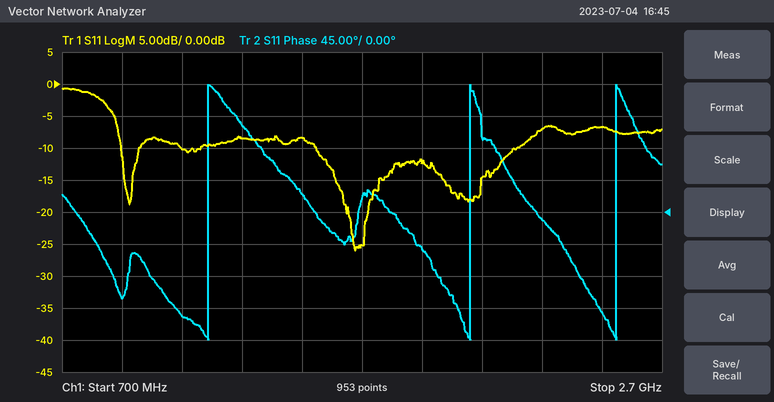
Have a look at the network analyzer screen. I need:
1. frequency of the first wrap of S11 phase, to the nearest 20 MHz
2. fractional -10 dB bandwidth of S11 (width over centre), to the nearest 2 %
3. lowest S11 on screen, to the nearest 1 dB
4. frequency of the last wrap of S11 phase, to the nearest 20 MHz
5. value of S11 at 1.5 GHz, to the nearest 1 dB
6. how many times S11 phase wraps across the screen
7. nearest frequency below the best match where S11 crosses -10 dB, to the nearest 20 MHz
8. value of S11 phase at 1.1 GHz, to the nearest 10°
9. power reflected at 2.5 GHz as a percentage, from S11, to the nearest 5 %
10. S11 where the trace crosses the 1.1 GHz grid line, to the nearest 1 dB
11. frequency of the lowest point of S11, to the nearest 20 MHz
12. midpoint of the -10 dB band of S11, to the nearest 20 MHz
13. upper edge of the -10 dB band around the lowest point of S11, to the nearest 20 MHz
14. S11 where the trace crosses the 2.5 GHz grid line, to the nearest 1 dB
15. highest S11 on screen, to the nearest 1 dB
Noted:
1.18 GHz
36 %
-26 dB
2.54 GHz
-8 dB
3
1.54 GHz
-150°
20 %
-10 dB
1.68 GHz
1.88 GHz
2.22 GHz
-7 dB
-1 dB
